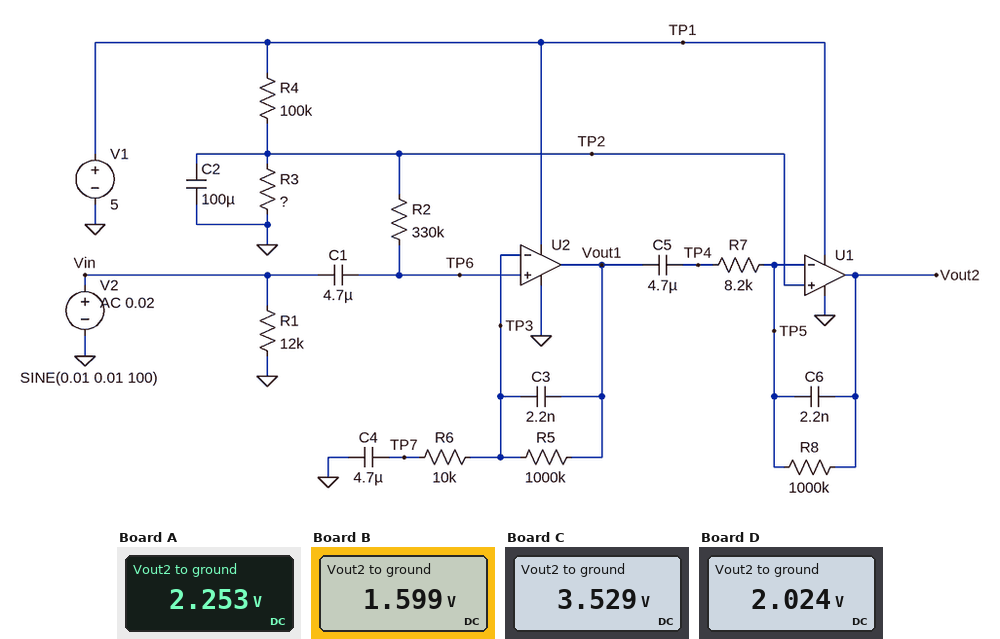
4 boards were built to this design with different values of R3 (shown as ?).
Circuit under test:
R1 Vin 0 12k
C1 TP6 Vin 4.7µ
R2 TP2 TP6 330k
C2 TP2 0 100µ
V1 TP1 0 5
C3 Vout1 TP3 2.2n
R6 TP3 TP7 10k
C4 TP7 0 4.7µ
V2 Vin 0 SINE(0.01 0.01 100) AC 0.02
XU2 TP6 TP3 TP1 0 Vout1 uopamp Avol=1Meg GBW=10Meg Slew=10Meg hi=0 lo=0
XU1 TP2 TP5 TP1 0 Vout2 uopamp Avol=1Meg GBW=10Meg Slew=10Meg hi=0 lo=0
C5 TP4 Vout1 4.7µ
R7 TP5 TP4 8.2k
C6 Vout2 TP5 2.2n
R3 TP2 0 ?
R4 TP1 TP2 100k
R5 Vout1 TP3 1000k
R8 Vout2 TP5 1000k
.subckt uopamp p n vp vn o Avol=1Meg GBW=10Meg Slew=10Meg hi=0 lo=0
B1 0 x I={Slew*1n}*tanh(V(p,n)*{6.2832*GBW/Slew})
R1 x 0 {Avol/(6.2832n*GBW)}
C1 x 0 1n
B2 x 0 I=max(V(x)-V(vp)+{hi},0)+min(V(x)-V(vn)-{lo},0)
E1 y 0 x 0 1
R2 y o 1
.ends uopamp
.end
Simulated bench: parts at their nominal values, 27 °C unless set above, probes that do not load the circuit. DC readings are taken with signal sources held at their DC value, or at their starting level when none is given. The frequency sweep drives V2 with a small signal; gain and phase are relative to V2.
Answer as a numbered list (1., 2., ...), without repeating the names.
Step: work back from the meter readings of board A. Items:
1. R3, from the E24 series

1. 82 kΩ
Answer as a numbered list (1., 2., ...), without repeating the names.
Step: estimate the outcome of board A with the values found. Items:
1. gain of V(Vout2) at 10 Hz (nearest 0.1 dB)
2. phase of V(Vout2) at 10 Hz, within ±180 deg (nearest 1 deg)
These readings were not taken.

1. 80.5 dB
2. -154 deg
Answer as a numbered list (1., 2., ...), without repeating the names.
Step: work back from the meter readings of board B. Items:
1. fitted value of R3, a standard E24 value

1. 47 kΩ
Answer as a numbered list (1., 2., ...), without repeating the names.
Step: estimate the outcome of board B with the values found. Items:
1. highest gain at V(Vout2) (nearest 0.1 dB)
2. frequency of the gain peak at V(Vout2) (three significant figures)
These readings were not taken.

1. 80.9 dB
2. 16.5 Hz
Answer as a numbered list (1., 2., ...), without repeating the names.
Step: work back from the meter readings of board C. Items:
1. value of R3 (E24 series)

1. 240 kΩ
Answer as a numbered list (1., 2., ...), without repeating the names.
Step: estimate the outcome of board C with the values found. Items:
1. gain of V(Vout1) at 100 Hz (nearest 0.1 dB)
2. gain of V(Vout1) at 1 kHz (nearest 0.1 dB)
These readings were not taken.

1. 35.4 dB
2. 17.3 dB
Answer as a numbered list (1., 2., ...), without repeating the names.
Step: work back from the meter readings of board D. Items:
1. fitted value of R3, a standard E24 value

1. 68 kΩ
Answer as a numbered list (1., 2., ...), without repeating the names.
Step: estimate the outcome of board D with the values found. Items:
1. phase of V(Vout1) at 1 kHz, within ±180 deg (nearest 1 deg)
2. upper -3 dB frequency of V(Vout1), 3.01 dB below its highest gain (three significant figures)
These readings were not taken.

1. -78 deg
2. 78.8 Hz
